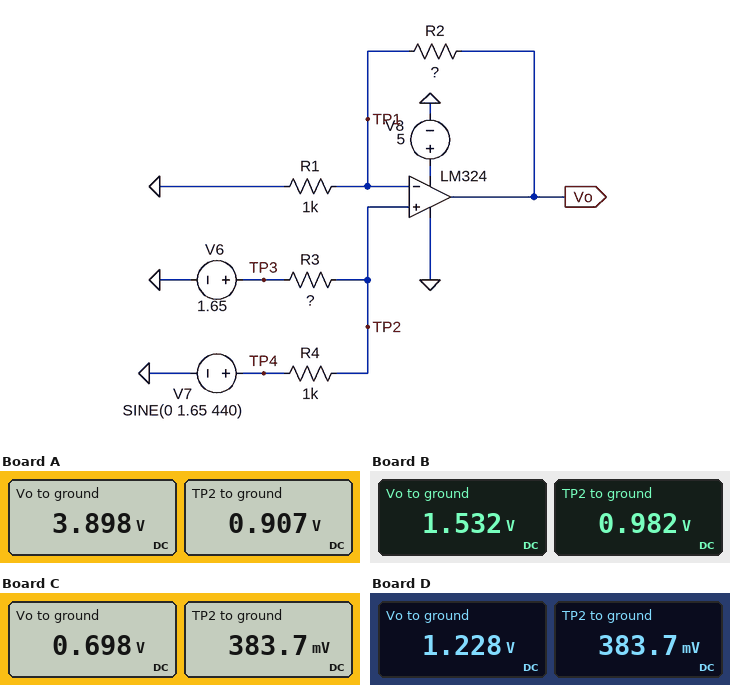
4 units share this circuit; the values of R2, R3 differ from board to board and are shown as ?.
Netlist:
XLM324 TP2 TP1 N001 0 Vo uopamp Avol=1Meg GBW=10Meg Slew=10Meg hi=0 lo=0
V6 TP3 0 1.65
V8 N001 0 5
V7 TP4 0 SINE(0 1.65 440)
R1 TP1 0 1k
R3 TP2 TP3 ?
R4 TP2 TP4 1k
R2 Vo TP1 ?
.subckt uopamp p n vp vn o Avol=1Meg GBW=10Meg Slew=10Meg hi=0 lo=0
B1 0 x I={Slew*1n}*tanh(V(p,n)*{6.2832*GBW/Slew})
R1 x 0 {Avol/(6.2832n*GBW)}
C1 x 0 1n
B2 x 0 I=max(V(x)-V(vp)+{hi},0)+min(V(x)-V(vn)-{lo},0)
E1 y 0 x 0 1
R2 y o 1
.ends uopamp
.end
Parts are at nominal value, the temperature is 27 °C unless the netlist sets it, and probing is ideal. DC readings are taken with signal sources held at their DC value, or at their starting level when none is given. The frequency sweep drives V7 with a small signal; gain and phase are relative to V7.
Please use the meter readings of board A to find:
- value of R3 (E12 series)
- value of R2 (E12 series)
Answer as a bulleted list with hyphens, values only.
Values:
- 820 Ω
- 3.3 kΩ
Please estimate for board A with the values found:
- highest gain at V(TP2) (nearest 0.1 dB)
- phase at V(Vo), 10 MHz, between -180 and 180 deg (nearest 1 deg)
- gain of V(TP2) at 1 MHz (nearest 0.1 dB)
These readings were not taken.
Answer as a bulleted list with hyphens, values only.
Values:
- -6.9 dB
- -77 deg
- -6.9 dB
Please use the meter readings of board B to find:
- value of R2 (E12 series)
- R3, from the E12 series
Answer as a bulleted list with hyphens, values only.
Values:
- 560 Ω
- 680 Ω
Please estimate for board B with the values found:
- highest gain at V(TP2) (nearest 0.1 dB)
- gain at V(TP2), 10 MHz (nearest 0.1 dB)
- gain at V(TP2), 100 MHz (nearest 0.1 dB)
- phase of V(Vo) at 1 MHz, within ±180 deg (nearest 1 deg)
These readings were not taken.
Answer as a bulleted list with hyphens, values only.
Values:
- -7.9 dB
- -7.9 dB
- -7.9 dB
- -9 deg
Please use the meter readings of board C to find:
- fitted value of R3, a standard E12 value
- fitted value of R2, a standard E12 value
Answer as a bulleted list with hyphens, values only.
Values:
- 3.3 kΩ
- 820 Ω
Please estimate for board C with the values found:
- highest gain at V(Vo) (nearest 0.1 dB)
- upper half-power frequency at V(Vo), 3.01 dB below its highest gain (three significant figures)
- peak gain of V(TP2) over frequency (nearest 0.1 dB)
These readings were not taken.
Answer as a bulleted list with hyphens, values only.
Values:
- 2.9 dB
- 5.49 MHz
- -2.3 dB
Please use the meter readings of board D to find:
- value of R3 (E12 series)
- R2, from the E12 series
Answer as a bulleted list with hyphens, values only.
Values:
- 3.3 kΩ
- 2.2 kΩ
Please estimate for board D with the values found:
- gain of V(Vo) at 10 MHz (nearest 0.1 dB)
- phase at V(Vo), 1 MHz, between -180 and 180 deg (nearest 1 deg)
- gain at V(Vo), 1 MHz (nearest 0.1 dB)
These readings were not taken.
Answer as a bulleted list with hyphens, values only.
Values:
- -2.7 dB
- -18 deg
- 7.4 dB
